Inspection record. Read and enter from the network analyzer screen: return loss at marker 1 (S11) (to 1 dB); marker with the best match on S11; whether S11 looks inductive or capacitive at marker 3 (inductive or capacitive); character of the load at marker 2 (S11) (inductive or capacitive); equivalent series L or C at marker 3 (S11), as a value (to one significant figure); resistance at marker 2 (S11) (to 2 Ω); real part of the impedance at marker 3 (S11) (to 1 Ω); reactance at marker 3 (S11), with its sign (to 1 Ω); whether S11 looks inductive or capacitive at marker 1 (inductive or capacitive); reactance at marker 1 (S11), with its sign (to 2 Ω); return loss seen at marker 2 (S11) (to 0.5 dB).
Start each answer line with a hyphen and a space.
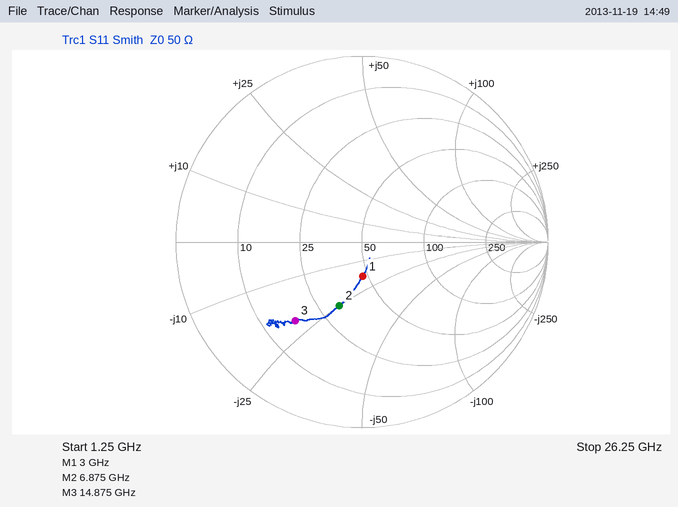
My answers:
- 15 dB
- marker 1
- capacitive
- capacitive
- 500 fF
- 32 Ω
- 17 Ω
- -21 Ω
- capacitive
- -18 Ω
- 9.0 dB
